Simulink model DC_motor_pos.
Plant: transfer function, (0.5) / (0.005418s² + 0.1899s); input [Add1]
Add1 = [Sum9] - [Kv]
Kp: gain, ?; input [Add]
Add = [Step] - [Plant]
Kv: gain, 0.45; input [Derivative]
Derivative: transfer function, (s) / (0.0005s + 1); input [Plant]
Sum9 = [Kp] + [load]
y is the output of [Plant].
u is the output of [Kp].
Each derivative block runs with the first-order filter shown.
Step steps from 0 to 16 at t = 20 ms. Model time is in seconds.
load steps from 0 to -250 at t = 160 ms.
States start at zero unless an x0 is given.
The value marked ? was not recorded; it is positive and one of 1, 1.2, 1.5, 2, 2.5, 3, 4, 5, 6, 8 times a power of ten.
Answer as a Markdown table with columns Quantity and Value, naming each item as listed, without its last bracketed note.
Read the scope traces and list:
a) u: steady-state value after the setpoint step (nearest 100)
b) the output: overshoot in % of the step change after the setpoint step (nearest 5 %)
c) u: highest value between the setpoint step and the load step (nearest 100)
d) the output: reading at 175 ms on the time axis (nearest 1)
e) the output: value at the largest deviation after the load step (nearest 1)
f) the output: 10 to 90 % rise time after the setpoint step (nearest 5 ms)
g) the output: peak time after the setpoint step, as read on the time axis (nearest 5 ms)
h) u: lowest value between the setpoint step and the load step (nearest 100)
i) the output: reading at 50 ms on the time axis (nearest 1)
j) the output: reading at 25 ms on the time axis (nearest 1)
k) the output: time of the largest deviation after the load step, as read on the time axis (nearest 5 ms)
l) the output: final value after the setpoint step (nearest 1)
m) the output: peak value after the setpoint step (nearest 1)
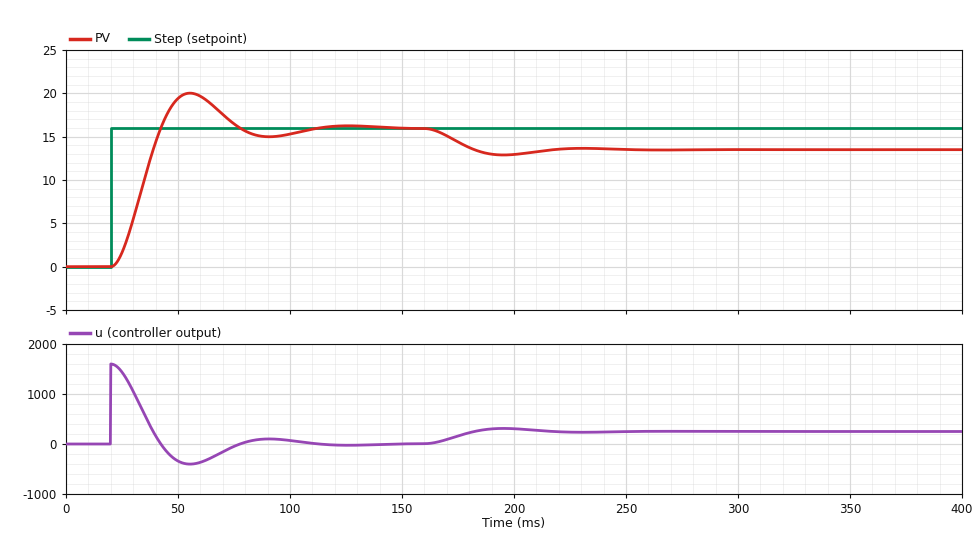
| Quantity | Value |
|---|---|
| u: steady-state value after the setpoint step | 0 |
| the output: overshoot in % of the step change after the setpoint step | 25 % |
| u: highest value between the setpoint step and the load step | 1600 |
| the output: reading at 175 ms on the time axis | 14 |
| the output: value at the largest deviation after the load step | 13 |
| the output: 10 to 90 % rise time after the setpoint step | 15 ms |
| the output: peak time after the setpoint step, as read on the time axis | 55 ms |
| u: lowest value between the setpoint step and the load step | -400 |
| the output: reading at 50 ms on the time axis | 19 |
| the output: reading at 25 ms on the time axis | 2 |
| the output: time of the largest deviation after the load step, as read on the time axis | 195 ms |
| the output: final value after the setpoint step | 16 |
| the output: peak value after the setpoint step | 20 |
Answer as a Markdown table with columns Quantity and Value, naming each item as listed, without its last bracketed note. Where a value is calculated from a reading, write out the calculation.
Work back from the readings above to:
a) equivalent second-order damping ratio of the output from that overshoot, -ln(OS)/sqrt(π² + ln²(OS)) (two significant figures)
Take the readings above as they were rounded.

| Quantity | Value |
|---|---|
| equivalent second-order damping ratio of the output from that overshoot, -ln(OS)/sqrt(π² + ln²(OS)) | ln(0.25) = -1.386; 1.386 / sqrt(9.870 + 1.922) = 0.40 |
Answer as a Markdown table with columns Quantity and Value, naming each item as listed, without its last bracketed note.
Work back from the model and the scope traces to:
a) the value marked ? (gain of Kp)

| Quantity | Value |
|---|---|
| the value marked ? | 100 |
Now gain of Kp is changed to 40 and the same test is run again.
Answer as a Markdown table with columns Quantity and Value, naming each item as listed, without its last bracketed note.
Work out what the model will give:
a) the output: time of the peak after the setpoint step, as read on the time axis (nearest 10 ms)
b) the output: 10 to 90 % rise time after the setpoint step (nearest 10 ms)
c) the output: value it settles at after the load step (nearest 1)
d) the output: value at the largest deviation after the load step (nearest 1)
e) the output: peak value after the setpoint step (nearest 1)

| Quantity | Value |
|---|---|
| the output: time of the peak after the setpoint step, as read on the time axis | 90 ms |
| the output: 10 to 90 % rise time after the setpoint step | 30 ms |
| the output: value it settles at after the load step | 10 |
| the output: value at the largest deviation after the load step | 9 |
| the output: peak value after the setpoint step | 17 |
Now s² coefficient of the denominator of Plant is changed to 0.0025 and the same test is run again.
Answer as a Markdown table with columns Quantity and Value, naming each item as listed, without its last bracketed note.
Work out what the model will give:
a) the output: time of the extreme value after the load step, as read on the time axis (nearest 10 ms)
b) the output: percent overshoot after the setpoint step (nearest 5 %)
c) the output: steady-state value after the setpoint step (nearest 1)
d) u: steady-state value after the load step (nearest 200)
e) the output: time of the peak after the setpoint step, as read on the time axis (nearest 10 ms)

| Quantity | Value |
|---|---|
| the output: time of the extreme value after the load step, as read on the time axis | 190 ms |
| the output: percent overshoot after the setpoint step | 10 % |
| the output: steady-state value after the setpoint step | 16 |
| u: steady-state value after the load step | 200 |
| the output: time of the peak after the setpoint step, as read on the time axis | 50 ms |
